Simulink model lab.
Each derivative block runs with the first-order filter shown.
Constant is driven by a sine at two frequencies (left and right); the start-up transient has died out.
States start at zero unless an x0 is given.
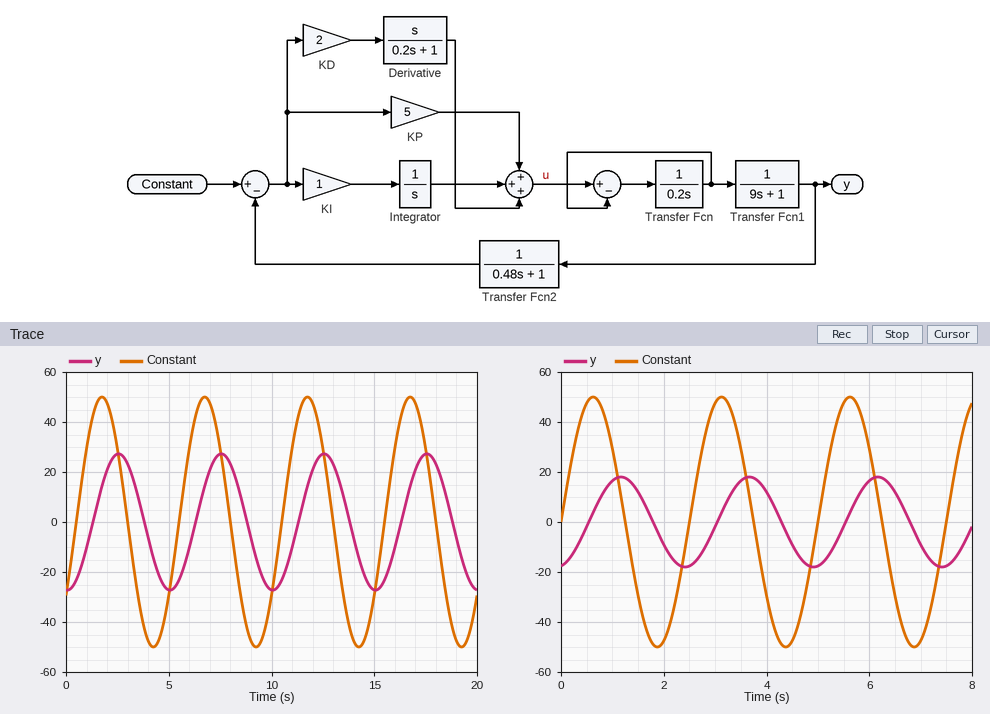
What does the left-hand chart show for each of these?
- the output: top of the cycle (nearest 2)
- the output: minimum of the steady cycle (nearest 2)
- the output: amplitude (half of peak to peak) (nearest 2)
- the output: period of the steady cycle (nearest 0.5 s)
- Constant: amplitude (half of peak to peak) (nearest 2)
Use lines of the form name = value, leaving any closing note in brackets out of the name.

the output: top of the cycle = 28
the output: minimum of the steady cycle = -28
the output: amplitude (half of peak to peak) = 28
the output: period of the steady cycle = 5.0 s
Constant: amplitude (half of peak to peak) = 50
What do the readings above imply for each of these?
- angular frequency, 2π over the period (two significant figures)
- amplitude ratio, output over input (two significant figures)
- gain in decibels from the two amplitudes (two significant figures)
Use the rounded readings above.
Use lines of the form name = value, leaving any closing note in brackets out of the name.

angular frequency, 2π over the period = 1.3 rad/s
amplitude ratio, output over input = 0.56
gain in decibels from the two amplitudes = -5.0 dB
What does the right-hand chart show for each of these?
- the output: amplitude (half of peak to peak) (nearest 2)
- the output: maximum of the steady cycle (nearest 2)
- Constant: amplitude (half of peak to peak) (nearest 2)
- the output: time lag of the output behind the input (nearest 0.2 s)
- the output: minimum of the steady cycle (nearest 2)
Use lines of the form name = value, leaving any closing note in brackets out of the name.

the output: amplitude (half of peak to peak) = 18
the output: maximum of the steady cycle = 18
Constant: amplitude (half of peak to peak) = 50
the output: time lag of the output behind the input = 0.6 s
the output: minimum of the steady cycle = -18
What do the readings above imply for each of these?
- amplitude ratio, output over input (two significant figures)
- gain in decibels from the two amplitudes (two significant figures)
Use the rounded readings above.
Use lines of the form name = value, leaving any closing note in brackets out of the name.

amplitude ratio, output over input = 0.36
gain in decibels from the two amplitudes = -8.9 dB
